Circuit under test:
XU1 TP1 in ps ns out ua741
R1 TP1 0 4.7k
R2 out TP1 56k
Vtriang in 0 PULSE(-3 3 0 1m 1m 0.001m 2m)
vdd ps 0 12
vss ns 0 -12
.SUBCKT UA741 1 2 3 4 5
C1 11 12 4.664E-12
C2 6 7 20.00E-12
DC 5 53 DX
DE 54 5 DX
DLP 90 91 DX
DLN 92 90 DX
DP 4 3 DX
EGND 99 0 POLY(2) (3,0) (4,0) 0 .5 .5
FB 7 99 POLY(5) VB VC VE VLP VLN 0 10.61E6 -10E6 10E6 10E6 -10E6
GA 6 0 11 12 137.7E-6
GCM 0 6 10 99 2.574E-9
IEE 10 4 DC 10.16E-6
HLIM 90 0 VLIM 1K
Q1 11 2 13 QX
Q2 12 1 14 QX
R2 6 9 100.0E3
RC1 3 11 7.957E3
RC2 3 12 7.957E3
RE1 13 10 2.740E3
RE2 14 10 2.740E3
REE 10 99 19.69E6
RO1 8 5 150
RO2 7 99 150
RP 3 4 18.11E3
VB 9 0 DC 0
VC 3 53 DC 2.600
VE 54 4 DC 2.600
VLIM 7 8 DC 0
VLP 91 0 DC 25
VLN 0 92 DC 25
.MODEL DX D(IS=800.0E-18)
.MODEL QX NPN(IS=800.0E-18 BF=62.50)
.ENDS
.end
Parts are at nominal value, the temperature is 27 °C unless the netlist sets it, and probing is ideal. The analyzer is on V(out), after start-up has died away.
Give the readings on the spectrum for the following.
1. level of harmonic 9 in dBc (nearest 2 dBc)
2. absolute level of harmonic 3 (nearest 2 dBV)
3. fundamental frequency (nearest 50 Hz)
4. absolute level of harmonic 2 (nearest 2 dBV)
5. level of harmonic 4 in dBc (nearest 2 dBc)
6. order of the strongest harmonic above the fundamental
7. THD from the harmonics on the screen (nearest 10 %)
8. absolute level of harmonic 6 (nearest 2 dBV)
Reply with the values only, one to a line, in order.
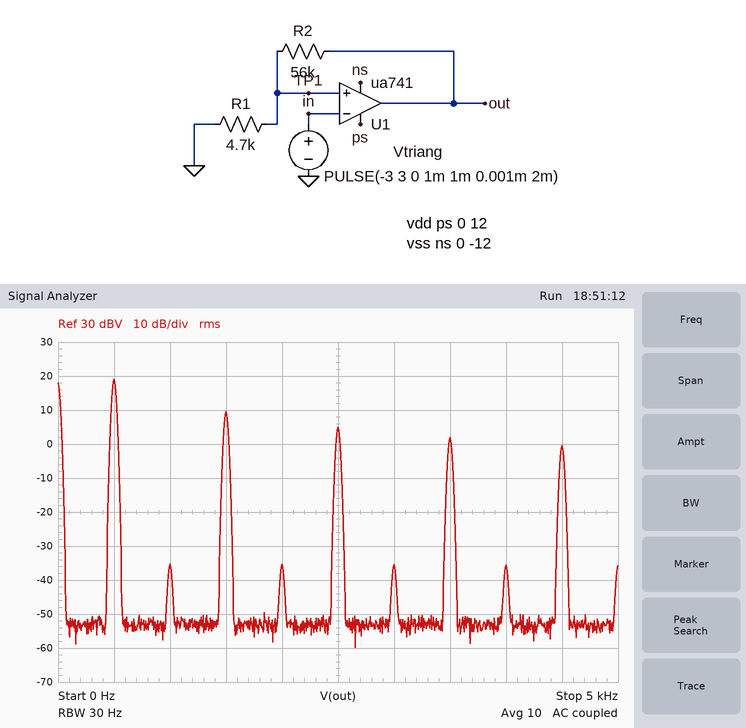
-20 dBc
10 dBV
500 Hz
-36 dBV
-54 dBc
3
40 %
-36 dBV
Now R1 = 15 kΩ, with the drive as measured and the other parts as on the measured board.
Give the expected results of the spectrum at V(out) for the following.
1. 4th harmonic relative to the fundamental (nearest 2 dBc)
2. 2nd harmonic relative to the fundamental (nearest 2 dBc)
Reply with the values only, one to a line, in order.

-52 dBc
-52 dBc
